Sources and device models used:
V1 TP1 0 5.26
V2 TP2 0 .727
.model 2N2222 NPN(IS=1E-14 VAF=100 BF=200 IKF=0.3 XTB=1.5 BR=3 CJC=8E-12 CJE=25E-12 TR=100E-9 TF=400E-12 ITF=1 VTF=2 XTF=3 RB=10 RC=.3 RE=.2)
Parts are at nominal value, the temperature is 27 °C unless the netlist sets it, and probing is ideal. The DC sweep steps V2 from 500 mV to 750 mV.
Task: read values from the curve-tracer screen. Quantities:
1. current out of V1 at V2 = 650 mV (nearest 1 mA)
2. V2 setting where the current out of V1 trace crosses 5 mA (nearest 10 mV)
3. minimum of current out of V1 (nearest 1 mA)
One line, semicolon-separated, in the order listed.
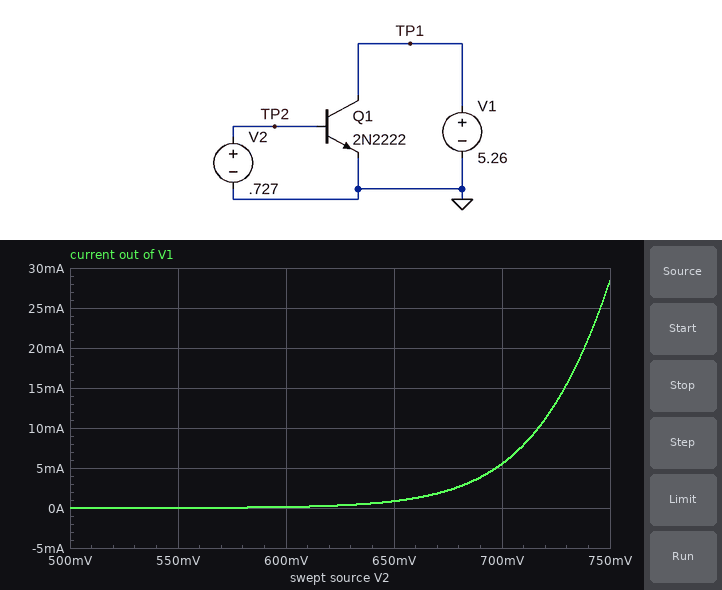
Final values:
1 mA; 700 mV; 0 A
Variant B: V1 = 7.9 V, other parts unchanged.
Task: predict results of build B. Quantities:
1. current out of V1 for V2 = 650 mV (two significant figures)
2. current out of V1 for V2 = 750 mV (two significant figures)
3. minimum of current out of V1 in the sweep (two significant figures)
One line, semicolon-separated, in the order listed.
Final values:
870 µA; 29 mA; 2.7 µA
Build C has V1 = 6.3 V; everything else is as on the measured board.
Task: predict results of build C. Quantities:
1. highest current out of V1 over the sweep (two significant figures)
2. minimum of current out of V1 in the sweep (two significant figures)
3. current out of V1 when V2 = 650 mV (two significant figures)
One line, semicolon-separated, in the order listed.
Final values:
29 mA; 2.6 µA; 860 µA
